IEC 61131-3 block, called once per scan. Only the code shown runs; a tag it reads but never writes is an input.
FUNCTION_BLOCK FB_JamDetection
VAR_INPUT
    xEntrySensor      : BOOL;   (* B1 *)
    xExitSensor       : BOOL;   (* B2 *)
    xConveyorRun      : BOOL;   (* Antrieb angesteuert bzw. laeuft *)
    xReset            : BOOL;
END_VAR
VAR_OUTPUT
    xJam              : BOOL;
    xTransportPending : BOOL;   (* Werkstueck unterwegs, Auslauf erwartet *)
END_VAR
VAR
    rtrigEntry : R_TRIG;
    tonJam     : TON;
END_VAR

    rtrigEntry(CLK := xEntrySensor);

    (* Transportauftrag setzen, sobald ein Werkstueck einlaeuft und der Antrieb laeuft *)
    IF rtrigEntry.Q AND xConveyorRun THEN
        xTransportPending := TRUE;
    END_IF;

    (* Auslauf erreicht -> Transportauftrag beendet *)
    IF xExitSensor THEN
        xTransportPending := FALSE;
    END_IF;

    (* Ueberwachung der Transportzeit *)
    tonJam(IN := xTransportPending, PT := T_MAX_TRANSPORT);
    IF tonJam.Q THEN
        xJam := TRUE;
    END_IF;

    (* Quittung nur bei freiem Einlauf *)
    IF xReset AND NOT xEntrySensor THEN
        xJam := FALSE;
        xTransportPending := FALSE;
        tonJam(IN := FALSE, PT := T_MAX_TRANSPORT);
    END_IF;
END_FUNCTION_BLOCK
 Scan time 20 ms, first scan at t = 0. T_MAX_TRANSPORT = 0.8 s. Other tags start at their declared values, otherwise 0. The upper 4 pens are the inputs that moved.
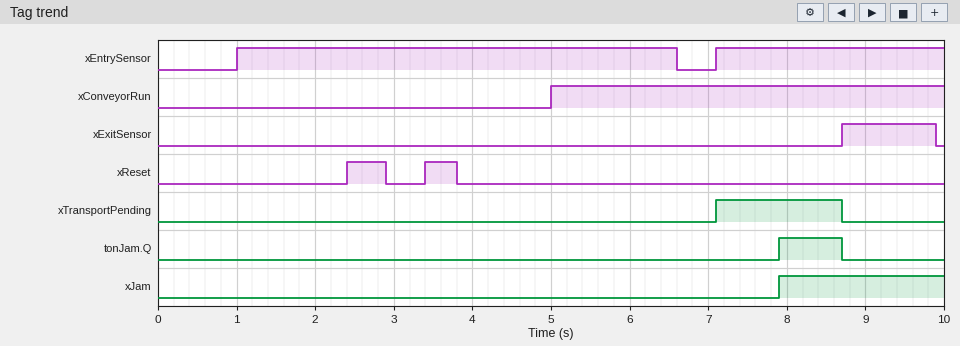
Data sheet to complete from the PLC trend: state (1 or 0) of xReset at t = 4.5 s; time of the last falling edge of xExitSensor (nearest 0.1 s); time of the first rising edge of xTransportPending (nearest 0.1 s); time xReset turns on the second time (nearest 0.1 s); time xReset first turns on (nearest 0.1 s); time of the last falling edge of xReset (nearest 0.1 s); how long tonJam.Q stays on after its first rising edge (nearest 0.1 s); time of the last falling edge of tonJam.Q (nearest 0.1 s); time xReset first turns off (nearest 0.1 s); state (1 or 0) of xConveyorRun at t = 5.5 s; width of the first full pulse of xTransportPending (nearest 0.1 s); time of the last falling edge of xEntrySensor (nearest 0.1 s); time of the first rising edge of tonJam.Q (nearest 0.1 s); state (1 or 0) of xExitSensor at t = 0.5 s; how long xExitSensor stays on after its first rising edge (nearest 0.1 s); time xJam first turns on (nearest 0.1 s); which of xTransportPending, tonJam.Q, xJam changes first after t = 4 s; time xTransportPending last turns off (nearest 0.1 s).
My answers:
0
9.9 s
7.1 s
3.4 s
2.4 s
3.8 s
0.8 s
8.7 s
2.9 s
1
1.6 s
6.6 s
7.9 s
0
1.2 s
7.9 s
xTransportPending
8.7 s
